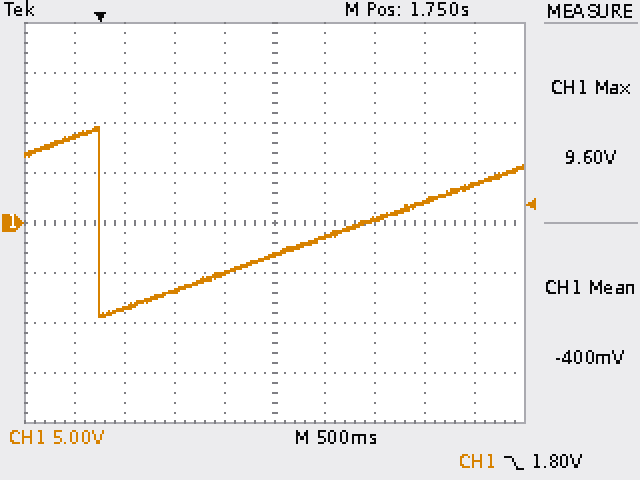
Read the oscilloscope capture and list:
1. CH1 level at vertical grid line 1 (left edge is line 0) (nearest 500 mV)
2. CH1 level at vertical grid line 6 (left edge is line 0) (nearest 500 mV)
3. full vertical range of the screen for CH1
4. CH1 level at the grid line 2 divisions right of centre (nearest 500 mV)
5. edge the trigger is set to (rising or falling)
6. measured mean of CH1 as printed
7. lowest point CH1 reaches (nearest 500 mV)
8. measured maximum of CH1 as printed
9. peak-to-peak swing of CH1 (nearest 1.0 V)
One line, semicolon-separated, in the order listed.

8.5 V; -1.5 V; 40 V; 500 mV; falling; -400 mV; -9.5 V; 9.60 V; 19.0 V
